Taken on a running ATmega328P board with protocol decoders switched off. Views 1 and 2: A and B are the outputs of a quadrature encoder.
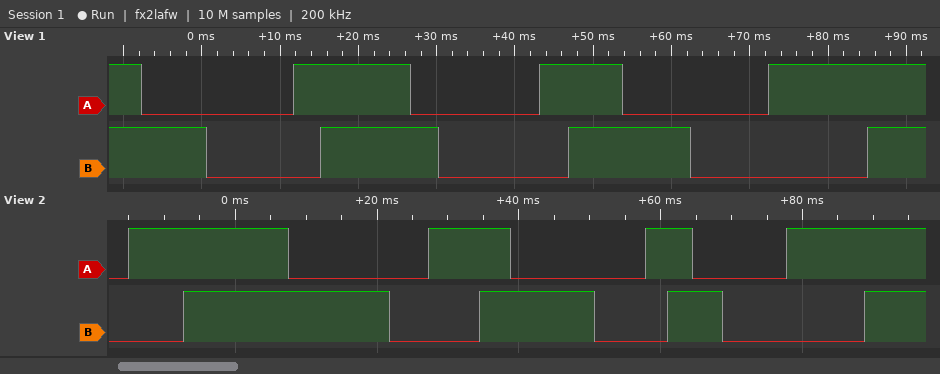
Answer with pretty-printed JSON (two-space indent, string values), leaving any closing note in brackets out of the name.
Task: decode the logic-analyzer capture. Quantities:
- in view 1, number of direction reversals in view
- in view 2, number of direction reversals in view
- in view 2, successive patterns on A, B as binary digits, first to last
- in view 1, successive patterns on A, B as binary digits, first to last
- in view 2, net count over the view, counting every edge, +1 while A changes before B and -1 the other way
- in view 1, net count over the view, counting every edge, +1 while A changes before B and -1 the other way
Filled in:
{
  "in view 1, number of direction reversals in view": "0",
  "in view 2, number of direction reversals in view": "0",
  "in view 2, successive patterns on A, B as binary digits, first to last": "00 10 11 01 00 10 11 01 00 10 11 01 00 10 11",
  "in view 1, successive patterns on A, B as binary digits, first to last": "11 01 00 10 11 01 00 10 11 01 00 10 11",
  "in view 2, net count over the view, counting every edge, +1 while A changes before B and -1 the other way": "+14",
  "in view 1, net count over the view, counting every edge, +1 while A changes before B and -1 the other way": "+12"
}
